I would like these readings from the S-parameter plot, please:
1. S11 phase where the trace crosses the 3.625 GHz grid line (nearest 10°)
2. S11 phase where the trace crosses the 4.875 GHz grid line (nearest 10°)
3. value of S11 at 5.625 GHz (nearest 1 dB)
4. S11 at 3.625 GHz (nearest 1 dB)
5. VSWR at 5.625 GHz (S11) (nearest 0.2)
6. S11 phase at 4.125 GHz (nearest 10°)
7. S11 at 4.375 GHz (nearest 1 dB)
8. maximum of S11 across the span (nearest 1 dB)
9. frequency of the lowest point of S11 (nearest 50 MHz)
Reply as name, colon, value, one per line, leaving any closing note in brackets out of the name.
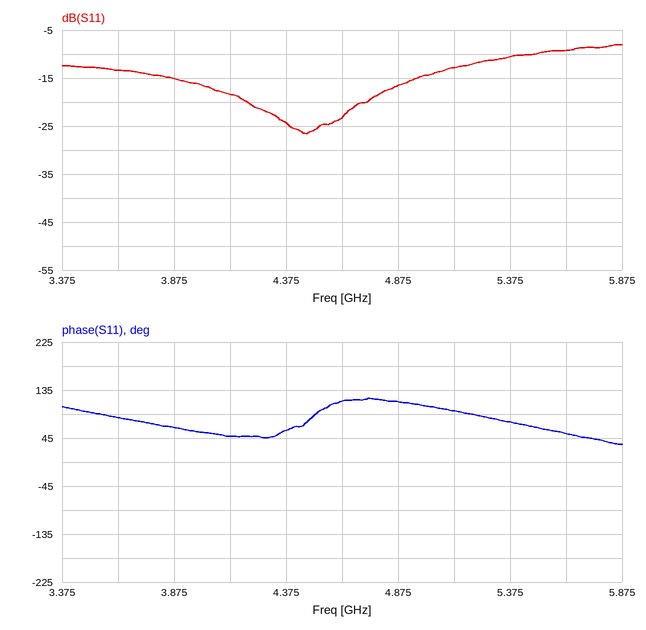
S11 phase where the trace crosses the 3.625 GHz grid line: 80°
S11 phase where the trace crosses the 4.875 GHz grid line: 110°
value of S11 at 5.625 GHz: -9 dB
S11 at 3.625 GHz: -13 dB
VSWR at 5.625 GHz (S11): 2.0
S11 phase at 4.125 GHz: 50°
S11 at 4.375 GHz: -24 dB
maximum of S11 across the span: -8 dB
frequency of the lowest point of S11: 4.45 GHz
